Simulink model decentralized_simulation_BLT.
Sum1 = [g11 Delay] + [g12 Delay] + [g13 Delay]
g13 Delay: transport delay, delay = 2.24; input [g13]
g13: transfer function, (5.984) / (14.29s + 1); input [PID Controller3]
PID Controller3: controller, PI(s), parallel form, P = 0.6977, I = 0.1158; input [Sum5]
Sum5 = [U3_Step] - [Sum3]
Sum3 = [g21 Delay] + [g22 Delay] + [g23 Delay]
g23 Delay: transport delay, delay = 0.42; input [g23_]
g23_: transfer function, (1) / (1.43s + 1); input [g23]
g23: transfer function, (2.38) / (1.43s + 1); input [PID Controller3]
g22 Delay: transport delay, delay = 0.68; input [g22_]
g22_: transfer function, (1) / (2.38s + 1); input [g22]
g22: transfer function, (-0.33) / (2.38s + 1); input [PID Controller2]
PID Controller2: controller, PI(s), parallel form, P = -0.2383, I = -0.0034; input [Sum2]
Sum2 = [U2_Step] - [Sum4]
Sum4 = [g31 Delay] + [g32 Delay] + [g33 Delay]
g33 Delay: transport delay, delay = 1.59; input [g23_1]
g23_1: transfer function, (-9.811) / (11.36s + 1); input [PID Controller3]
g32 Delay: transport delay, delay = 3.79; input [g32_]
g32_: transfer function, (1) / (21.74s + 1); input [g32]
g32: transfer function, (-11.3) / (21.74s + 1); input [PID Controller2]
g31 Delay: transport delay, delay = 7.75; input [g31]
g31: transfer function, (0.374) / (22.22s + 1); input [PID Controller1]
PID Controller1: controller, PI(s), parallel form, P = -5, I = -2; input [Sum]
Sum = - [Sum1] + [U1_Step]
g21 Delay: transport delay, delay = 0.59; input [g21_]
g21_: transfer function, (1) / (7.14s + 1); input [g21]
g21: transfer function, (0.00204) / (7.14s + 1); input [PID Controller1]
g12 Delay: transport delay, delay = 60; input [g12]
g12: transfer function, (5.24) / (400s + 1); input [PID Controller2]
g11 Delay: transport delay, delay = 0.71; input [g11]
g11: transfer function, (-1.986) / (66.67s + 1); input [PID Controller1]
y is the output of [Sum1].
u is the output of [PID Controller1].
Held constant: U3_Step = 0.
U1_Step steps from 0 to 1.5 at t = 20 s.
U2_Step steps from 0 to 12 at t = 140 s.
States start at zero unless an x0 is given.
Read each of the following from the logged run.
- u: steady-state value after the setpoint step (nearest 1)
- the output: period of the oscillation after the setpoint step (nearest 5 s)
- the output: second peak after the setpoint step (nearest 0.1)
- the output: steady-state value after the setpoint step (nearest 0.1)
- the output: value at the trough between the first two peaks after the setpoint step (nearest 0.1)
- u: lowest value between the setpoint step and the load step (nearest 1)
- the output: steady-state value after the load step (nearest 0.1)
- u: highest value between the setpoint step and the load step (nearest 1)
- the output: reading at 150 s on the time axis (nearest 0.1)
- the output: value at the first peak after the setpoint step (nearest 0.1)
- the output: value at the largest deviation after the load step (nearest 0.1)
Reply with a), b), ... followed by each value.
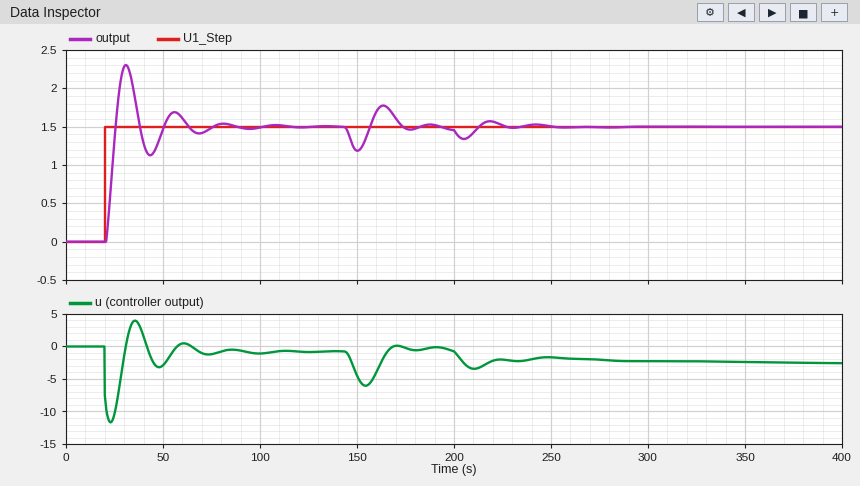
a) -1
b) 25 s
c) 1.7
d) 1.5
e) 1.1
f) -12
g) 1.5
h) 4
i) 1.2
j) 2.3
k) 1.2
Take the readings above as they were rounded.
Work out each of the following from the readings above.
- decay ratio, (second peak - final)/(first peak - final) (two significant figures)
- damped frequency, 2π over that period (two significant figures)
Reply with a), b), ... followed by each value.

a) 0.25
b) 0.25 rad/s
